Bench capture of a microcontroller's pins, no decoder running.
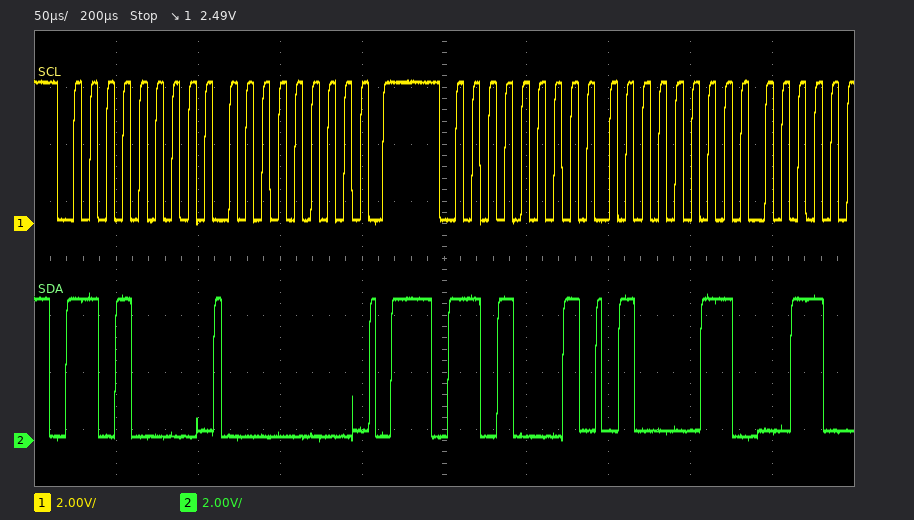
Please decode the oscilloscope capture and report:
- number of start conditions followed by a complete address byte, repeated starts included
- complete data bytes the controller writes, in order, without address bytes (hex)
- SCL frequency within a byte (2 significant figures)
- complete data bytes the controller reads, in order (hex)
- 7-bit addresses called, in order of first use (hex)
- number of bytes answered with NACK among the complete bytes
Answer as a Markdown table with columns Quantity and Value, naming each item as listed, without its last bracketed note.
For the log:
| Quantity | Value |
|---|---|
| number of start conditions followed by a complete address byte, repeated starts included | 2 |
| complete data bytes the controller writes, in order, without address bytes | 00 |
| SCL frequency within a byte | 100 kHz |
| complete data bytes the controller reads, in order | 43 |
| 7-bit addresses called, in order of first use | 0x68 |
| number of bytes answered with NACK among the complete bytes | 0 |
